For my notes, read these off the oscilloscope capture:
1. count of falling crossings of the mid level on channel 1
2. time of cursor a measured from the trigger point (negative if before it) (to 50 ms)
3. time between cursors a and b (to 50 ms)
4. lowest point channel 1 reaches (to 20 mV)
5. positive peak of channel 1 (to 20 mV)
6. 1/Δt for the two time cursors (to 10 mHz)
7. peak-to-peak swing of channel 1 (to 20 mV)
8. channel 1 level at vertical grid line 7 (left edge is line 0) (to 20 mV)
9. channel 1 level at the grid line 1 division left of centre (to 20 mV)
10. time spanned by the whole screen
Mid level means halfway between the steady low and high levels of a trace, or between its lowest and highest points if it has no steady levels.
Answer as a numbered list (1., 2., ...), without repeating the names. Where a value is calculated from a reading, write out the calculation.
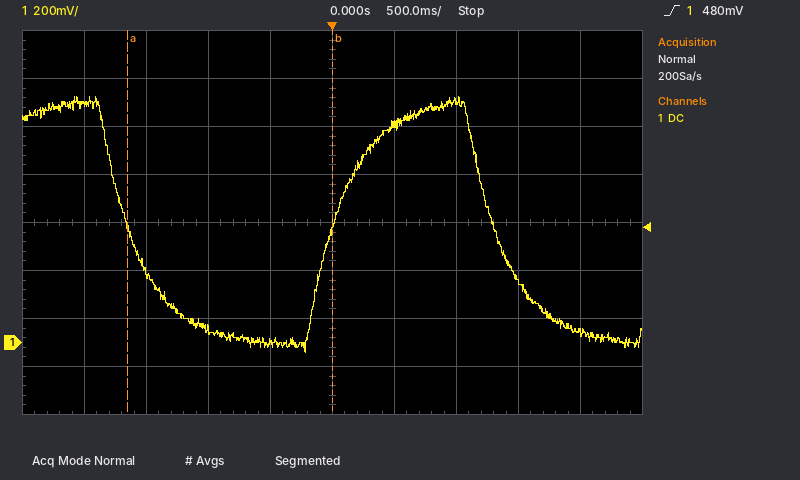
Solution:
1. 2
2. -1.65 s
3. 1.65 s
4. -40 mV
5. 1.02 V
6. 1 / 1.65 s ≈ 610 mHz
7. 1.02 V − (-40 mV) = 1.06 V
8. 1.00 V
9. 0 mV
10. 5 s
